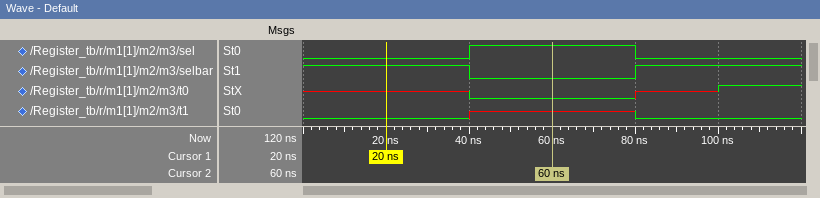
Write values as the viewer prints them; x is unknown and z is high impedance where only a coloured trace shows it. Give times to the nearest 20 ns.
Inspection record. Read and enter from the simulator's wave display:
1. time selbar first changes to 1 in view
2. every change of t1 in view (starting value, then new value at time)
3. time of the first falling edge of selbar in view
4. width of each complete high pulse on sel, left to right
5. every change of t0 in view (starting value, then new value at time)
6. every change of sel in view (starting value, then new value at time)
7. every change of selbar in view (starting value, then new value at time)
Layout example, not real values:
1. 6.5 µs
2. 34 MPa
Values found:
1. 80 ns
2. 0, x at 40 ns, 0 at 80 ns
3. 40 ns
4. 40 ns
5. x, 0 at 40 ns, x at 80 ns, 1 at 100 ns
6. 0, 1 at 40 ns, 0 at 80 ns
7. 1, 0 at 40 ns, 1 at 80 ns
